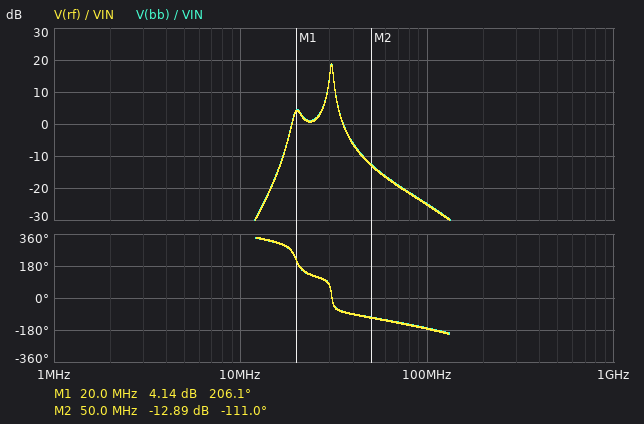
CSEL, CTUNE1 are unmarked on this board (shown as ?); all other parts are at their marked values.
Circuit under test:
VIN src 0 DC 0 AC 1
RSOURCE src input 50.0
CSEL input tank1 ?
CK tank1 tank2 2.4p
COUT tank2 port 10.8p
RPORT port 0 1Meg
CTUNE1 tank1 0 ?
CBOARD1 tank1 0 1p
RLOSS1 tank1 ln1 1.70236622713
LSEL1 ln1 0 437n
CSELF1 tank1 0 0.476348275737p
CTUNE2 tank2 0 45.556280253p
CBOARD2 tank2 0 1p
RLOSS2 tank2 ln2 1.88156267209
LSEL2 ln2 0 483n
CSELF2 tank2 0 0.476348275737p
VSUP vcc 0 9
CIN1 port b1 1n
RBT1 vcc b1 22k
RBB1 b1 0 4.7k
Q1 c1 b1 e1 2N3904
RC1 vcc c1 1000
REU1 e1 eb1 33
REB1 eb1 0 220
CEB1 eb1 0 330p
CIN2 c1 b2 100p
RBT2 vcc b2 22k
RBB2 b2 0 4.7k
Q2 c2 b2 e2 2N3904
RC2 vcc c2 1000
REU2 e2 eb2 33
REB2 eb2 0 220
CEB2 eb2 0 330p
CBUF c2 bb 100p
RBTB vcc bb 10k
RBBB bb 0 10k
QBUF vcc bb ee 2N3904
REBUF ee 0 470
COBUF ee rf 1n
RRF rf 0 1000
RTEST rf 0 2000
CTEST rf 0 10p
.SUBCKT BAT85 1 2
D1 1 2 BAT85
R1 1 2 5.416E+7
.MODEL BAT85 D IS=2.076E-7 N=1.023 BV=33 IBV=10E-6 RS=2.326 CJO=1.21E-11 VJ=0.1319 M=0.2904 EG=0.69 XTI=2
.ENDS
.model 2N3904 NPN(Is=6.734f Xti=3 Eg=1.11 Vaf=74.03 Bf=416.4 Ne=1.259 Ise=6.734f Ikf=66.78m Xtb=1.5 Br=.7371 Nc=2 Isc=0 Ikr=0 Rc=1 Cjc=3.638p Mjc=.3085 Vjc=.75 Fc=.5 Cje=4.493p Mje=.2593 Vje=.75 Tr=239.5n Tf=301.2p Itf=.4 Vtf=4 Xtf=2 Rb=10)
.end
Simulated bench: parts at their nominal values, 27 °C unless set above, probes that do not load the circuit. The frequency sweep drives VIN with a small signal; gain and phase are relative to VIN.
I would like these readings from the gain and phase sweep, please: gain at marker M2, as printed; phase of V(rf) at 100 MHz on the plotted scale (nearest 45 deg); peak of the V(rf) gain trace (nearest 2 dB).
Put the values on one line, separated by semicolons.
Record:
-12.89 dB; -180 deg; 18 dB
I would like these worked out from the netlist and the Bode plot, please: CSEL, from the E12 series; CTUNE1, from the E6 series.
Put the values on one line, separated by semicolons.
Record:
47 pF; 100 pF
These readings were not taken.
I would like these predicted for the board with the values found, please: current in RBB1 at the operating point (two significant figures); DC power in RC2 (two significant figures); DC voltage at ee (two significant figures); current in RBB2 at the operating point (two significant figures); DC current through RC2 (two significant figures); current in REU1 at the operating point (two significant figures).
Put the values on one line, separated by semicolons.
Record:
320 µA; 10 mW; 3.6 V; 320 µA; 3.2 mA; 3.2 mA
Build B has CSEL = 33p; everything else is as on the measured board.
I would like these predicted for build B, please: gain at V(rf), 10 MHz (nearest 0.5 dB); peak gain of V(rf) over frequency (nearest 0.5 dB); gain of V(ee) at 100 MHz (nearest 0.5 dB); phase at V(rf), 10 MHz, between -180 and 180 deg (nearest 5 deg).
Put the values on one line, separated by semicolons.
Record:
-41.5 dB; 17.0 dB; -26.5 dB; 0 deg
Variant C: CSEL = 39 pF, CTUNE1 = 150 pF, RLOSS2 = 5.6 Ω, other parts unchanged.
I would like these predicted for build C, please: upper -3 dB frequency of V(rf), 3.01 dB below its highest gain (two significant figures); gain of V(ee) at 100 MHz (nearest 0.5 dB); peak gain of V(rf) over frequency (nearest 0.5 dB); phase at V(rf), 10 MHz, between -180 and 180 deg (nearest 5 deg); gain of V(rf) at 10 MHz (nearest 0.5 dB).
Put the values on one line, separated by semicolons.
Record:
32 MHz; -29.0 dB; 7.5 dB; -10 deg; -38.5 dB
